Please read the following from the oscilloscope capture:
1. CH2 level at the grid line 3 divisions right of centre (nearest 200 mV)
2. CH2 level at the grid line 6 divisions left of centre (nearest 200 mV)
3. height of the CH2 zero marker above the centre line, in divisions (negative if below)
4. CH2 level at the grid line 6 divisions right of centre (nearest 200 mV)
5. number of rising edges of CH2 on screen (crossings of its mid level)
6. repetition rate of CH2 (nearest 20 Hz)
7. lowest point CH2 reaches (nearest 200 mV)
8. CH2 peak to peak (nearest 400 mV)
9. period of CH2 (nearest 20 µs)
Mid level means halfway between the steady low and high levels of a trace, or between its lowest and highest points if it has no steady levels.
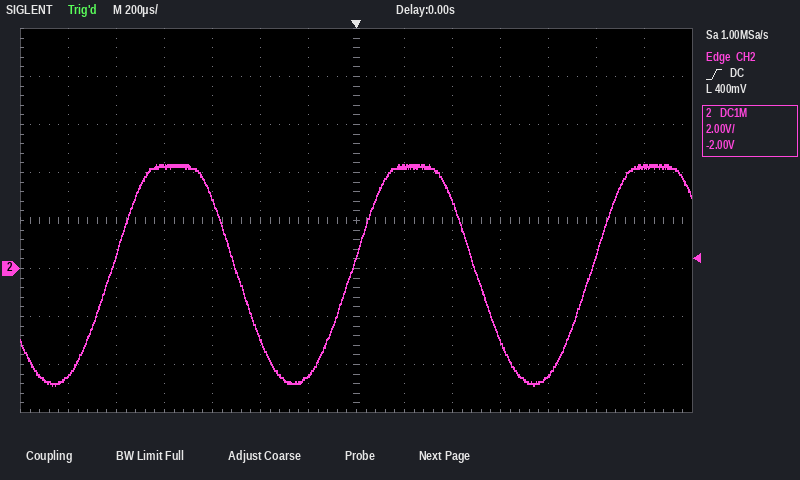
-3.0 V
-4.4 V
-1.0 div
4.2 V
3
1.00 kHz
-4.8 V
9.2 V
1.00 ms
